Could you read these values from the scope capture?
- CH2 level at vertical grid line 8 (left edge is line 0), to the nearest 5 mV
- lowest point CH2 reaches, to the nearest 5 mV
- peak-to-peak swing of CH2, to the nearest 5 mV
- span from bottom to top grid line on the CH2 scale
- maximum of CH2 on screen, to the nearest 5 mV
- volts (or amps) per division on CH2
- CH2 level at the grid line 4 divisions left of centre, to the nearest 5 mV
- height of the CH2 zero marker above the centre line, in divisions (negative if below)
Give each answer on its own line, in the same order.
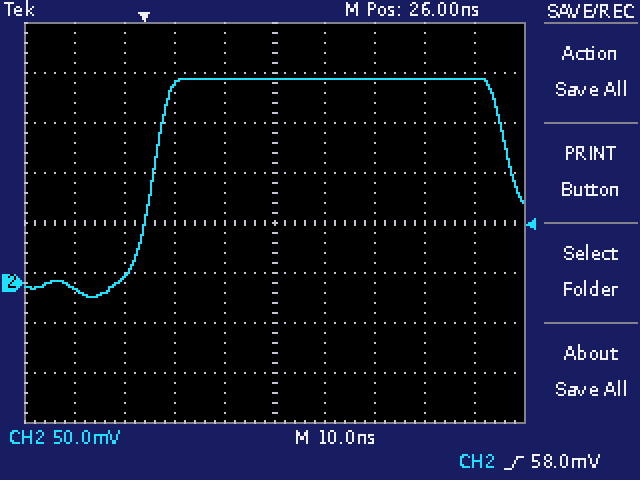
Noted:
205 mV
-15 mV
220 mV
400 mV
205 mV
50 mV
-5 mV
-1.2 div
